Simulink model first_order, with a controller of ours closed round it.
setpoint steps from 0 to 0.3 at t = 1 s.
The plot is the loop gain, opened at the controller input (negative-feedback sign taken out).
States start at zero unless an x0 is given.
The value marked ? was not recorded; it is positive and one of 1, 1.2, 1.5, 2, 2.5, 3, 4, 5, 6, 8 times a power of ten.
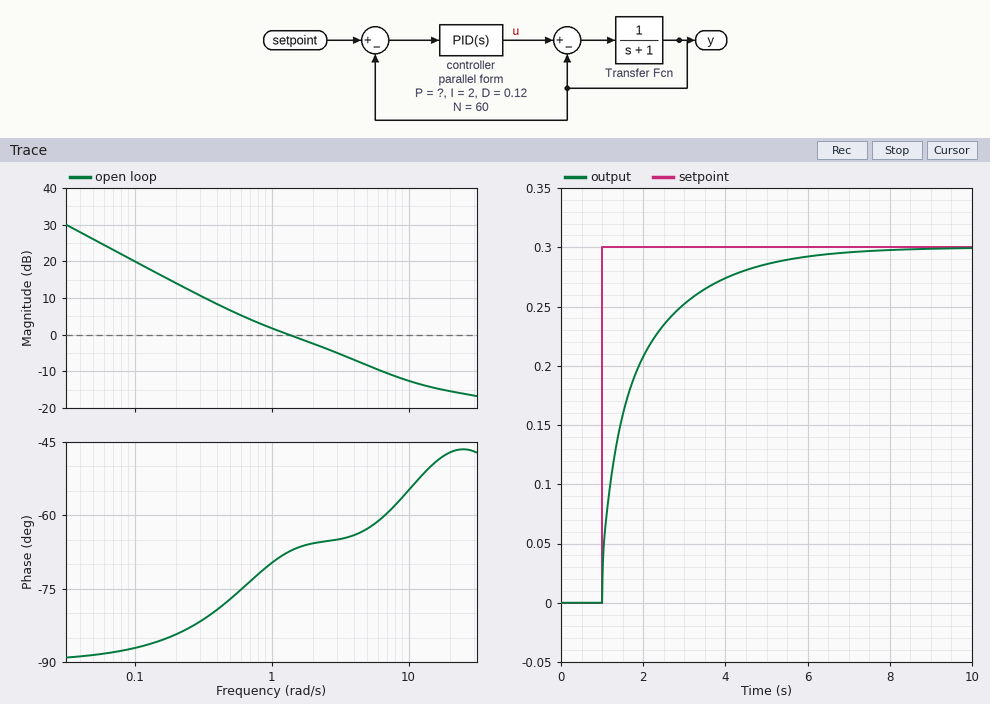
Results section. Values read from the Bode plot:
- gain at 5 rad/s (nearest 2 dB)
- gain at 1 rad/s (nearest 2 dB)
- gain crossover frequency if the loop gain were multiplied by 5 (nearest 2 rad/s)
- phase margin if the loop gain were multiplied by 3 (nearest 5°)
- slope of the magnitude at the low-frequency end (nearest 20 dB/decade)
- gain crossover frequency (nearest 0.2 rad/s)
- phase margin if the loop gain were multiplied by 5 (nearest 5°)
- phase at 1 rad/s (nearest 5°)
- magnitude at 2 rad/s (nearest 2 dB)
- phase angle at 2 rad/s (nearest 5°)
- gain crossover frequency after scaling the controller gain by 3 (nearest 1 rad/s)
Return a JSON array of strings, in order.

["-8 dB", "2 dB", "14 rad/s", "120°", "-20 dB/decade", "1.4 rad/s", "130°", "-70°", "-2 dB", "-65°", "6 rad/s"]
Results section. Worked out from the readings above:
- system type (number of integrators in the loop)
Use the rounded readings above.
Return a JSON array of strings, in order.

["1"]
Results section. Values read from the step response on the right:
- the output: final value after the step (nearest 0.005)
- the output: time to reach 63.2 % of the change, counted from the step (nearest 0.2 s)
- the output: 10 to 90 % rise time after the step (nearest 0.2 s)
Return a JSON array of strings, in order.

["0.300", "0.8 s", "2.8 s"]
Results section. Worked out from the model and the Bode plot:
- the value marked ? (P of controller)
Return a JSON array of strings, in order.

["2"]
